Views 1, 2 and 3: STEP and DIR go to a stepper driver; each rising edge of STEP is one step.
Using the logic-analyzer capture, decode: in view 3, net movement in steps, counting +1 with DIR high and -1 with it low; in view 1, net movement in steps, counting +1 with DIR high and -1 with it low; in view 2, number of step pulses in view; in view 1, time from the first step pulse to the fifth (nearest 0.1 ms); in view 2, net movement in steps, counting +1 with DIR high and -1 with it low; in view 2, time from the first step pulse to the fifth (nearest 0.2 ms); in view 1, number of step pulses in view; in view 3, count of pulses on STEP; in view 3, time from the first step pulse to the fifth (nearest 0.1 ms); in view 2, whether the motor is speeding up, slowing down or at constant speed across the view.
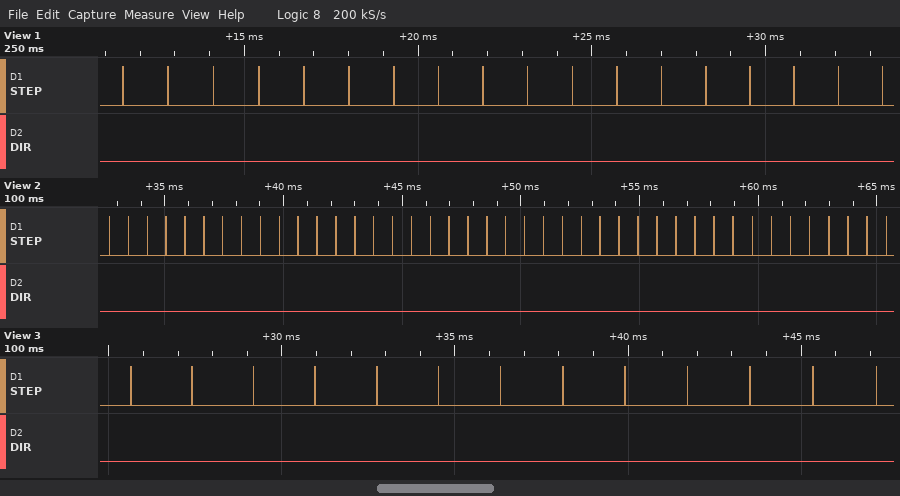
-13
-18
42
5.2 ms
-42
3.2 ms
18
13
7.1 ms
constant speed
